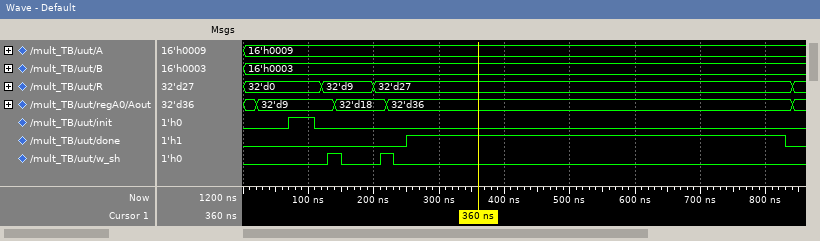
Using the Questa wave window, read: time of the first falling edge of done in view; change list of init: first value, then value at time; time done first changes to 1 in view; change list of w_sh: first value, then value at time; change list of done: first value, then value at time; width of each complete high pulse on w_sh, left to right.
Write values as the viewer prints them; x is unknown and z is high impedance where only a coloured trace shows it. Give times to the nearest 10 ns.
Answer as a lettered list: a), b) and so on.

a) 830 ns
b) 0, 1 at 70 ns, 0 at 110 ns
c) 250 ns
d) 0, 1 at 130 ns, 0 at 150 ns, 1 at 210 ns, 0 at 230 ns
e) 0, 1 at 250 ns, 0 at 830 ns
f) 20 ns, 20 ns
